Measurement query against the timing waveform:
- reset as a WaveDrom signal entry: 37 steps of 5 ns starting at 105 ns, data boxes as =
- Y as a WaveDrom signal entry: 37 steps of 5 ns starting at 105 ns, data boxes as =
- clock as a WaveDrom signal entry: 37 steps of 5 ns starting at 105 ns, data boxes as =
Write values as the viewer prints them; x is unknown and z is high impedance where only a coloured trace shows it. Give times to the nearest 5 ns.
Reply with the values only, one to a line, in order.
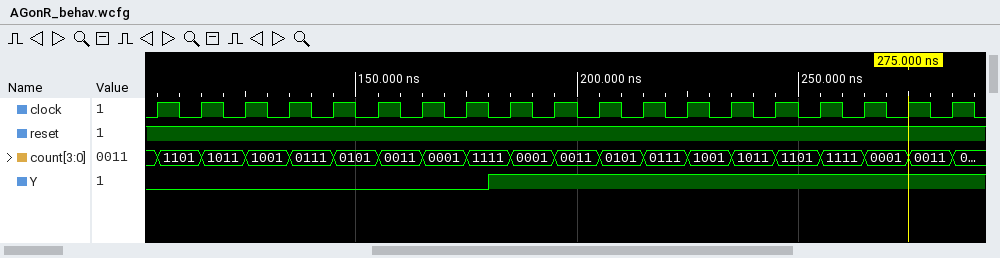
{name: 'reset', wave: '1....................................'}
{name: 'Y', wave: '0..............1.....................'}
{name: 'clock', wave: '1010101010101010101010101010101010101'}
